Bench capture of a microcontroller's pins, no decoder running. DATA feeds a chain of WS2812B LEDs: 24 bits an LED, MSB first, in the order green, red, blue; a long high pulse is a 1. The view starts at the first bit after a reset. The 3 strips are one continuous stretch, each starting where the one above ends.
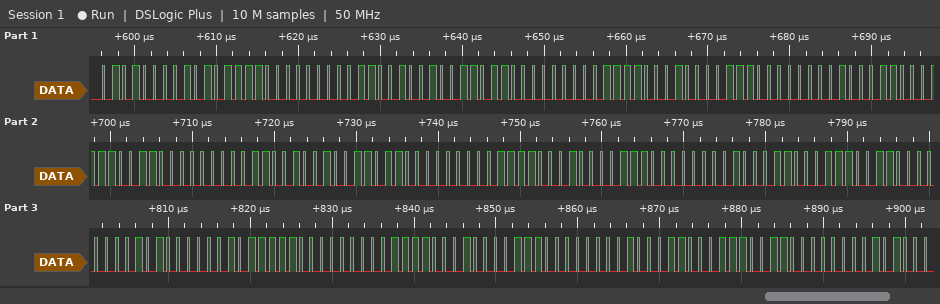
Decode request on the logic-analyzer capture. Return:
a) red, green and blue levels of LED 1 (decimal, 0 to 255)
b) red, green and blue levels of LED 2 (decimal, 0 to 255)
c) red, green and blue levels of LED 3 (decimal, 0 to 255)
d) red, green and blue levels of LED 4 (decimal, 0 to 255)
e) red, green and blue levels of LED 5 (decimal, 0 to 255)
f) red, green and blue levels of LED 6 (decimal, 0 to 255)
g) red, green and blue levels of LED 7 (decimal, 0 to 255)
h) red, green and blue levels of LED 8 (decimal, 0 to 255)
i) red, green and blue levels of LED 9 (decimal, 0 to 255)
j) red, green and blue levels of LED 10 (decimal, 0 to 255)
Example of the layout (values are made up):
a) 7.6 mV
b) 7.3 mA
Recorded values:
a) 175, 80, 0
b) 155, 100, 0
c) 135, 120, 0
d) 115, 140, 0
e) 155, 100, 0
f) 135, 120, 0
g) 115, 140, 0
h) 95, 160, 0
i) 135, 120, 0
j) 115, 140, 0
